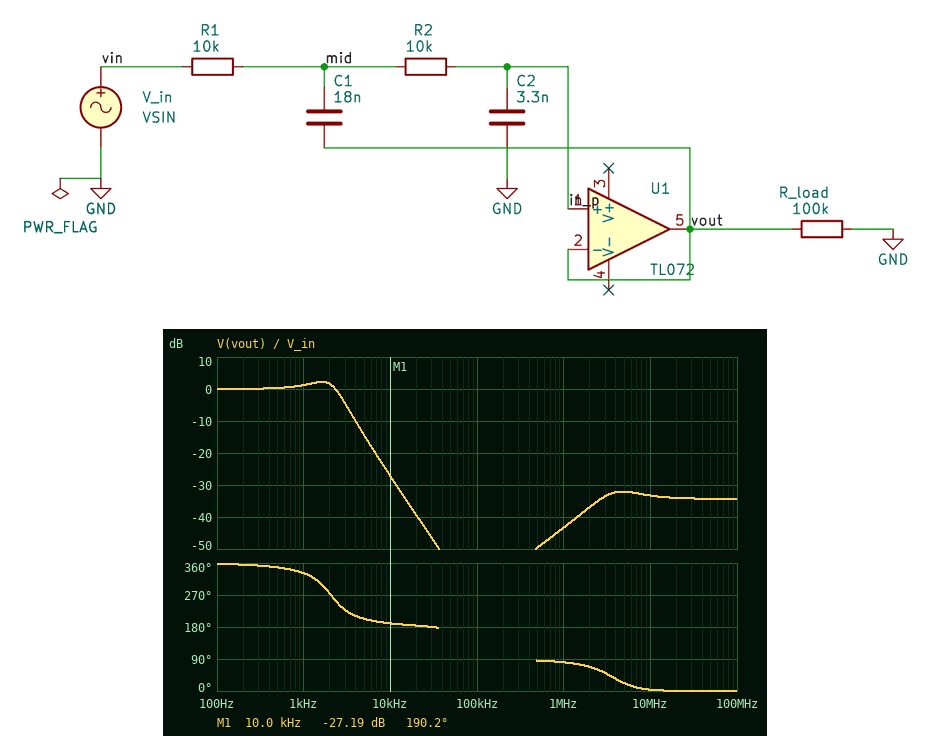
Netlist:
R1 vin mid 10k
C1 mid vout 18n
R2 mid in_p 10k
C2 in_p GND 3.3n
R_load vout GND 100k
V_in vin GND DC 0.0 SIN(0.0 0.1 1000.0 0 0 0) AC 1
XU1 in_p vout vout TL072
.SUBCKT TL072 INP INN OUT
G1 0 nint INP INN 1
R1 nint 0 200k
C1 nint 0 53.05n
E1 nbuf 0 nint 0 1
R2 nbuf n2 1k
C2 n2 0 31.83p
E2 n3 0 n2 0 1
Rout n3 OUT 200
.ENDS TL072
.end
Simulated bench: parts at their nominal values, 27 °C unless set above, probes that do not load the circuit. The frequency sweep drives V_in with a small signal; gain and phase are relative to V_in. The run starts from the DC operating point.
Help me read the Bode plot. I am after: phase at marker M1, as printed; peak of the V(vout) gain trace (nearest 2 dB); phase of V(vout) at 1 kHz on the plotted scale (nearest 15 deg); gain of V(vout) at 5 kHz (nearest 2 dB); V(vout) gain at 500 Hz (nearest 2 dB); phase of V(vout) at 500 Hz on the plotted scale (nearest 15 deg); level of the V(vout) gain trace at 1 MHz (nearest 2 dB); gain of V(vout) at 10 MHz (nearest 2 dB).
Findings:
190.2 deg
2 dB
330 deg
-14 dB
0 dB
345 deg
-44 dB
-34 dB
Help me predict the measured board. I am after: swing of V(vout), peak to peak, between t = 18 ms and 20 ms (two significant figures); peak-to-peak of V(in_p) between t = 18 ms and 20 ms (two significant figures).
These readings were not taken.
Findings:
230 mV
230 mV
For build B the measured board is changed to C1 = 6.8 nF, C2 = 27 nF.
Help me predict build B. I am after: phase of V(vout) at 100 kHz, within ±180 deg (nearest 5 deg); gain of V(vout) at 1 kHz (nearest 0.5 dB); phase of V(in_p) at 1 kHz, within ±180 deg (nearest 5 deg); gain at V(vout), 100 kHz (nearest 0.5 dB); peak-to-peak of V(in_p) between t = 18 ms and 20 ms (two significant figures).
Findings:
105 deg
-10.5 dB
-85 deg
-63.5 dB
59 mV
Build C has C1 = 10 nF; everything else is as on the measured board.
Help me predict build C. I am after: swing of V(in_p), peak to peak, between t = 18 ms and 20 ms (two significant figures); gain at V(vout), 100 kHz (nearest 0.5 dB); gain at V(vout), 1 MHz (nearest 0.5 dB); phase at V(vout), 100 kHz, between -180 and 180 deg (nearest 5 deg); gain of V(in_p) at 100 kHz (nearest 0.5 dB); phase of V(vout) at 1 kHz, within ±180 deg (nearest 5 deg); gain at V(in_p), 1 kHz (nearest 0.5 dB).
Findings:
210 mV
-60.0 dB
-43.5 dB
140 deg
-62.5 dB
-25 deg
0.5 dB
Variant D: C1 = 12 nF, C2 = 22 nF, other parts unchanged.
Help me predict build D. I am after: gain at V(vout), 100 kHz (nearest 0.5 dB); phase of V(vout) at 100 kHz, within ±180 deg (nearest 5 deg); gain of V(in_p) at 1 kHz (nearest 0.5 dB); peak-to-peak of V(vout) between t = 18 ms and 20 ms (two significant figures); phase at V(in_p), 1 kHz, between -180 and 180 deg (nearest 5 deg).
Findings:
-63.5 dB
100 deg
-9.0 dB
72 mV
-90 deg
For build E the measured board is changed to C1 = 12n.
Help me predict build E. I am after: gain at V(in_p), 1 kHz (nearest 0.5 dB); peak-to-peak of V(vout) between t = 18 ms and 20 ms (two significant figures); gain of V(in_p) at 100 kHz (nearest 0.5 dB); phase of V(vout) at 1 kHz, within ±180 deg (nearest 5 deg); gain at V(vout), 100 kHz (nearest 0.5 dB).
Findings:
0.5 dB
210 mV
-64.5 dB
-25 deg
-61.0 dB
